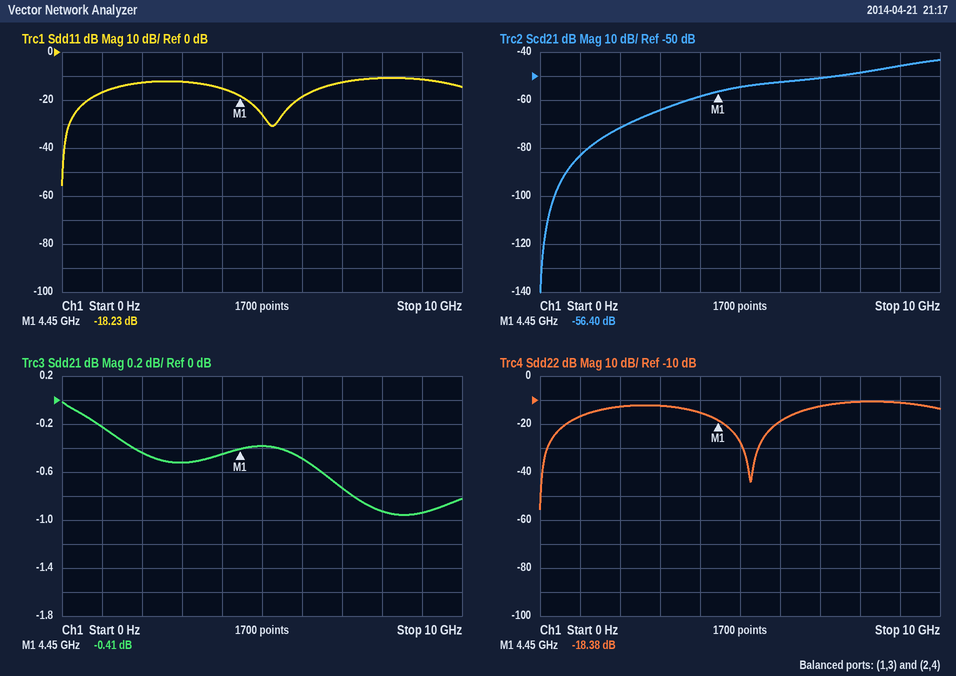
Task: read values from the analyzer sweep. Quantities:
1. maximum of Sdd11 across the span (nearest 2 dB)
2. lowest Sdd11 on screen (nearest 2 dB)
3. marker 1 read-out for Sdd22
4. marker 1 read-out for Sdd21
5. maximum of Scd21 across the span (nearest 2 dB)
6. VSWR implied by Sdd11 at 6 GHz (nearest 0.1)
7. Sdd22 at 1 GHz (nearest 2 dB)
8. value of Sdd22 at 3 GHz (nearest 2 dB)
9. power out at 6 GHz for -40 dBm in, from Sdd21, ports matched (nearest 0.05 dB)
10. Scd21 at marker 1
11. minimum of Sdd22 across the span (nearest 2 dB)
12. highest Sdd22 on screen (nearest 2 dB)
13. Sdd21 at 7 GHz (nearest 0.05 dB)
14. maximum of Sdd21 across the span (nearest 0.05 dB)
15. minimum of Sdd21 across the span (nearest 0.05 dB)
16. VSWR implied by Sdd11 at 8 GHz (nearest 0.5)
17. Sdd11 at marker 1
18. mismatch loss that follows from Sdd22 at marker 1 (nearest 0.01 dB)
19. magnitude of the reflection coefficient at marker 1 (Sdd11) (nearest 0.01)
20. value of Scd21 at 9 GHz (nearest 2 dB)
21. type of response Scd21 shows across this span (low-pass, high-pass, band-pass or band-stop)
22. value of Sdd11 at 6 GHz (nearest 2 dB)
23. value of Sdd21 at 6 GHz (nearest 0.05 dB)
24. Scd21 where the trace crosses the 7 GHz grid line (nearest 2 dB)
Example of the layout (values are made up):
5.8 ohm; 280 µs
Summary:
-10 dB; -56 dB; -18.38 dB; -0.41 dB; -44 dB; 1.3; -16 dB; -12 dB; -40.50 dBm; -56.40 dB; -56 dB; -10 dB; -0.75 dB; 0.00 dB; -0.95 dB; 2.0; -18.23 dB; 0.06 dB; 0.12; -46 dB; high-pass; -18 dB; -0.50 dB; -50 dB
